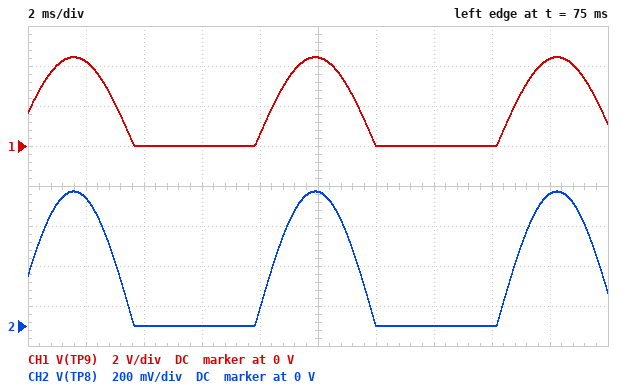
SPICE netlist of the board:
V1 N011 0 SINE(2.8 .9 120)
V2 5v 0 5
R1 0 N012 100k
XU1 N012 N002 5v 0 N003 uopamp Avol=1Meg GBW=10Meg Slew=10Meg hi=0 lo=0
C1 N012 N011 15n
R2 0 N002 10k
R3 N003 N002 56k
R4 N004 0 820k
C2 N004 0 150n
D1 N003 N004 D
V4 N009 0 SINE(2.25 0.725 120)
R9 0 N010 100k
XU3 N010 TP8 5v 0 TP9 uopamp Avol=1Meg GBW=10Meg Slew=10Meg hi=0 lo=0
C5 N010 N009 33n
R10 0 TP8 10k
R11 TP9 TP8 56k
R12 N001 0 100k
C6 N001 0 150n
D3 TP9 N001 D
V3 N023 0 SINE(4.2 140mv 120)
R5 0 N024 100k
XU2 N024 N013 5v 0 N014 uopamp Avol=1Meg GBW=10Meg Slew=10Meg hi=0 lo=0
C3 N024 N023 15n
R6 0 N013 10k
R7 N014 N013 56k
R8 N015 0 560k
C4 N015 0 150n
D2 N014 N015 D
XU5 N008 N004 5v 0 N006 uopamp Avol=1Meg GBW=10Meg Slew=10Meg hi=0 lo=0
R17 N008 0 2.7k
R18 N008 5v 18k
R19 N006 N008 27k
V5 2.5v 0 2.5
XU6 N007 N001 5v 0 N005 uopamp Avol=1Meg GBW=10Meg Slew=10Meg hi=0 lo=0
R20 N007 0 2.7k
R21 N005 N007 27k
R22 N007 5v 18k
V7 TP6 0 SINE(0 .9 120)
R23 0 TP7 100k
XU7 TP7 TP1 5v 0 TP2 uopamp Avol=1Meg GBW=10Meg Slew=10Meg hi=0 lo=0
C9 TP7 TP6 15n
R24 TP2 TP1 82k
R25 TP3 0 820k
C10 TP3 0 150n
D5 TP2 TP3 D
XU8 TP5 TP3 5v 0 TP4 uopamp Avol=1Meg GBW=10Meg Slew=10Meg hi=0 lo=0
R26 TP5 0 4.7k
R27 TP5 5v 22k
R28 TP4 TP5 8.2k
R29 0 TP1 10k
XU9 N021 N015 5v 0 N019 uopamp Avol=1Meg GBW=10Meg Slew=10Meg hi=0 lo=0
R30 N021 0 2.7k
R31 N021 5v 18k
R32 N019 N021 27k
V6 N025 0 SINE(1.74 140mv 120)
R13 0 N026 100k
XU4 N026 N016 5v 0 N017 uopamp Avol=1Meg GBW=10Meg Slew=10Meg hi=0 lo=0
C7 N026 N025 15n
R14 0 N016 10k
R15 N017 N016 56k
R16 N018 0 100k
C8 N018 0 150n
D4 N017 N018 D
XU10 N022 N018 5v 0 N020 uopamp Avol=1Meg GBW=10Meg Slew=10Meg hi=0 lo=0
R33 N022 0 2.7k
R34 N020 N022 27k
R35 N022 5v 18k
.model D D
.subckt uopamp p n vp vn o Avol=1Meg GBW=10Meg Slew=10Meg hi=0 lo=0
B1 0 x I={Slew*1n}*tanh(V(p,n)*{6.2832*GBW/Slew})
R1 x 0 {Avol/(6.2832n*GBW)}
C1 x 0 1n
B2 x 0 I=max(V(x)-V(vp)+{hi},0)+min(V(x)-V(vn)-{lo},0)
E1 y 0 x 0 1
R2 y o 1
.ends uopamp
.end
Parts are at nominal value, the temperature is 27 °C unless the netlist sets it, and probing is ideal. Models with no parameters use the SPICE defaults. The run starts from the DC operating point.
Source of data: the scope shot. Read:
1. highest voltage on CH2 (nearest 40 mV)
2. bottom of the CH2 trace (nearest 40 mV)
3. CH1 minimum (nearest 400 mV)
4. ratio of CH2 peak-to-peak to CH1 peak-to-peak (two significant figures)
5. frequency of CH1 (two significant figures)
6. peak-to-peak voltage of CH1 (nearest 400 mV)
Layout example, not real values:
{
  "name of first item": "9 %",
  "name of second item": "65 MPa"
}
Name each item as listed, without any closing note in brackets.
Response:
{
  "highest voltage on CH2": "680 mV",
  "bottom of the CH2 trace": "0 V",
  "CH1 minimum": "0 V",
  "ratio of CH2 peak-to-peak to CH1 peak-to-peak": "0.15",
  "frequency of CH1": "120 Hz",
  "peak-to-peak voltage of CH1": "4.4 V"
}
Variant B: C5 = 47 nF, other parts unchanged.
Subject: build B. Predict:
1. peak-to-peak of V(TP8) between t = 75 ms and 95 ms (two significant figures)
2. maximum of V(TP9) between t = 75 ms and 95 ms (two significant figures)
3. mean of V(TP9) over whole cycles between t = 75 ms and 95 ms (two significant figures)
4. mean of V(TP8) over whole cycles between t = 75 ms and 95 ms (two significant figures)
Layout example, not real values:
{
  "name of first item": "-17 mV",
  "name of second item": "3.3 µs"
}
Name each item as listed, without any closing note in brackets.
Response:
{
  "peak-to-peak of V(TP8) between t = 75 ms and 95 ms": "700 mV",
  "maximum of V(TP9) between t = 75 ms and 95 ms": "4.6 V",
  "mean of V(TP9) over whole cycles between t = 75 ms and 95 ms": "1.5 V",
  "mean of V(TP8) over whole cycles between t = 75 ms and 95 ms": "220 mV"
}
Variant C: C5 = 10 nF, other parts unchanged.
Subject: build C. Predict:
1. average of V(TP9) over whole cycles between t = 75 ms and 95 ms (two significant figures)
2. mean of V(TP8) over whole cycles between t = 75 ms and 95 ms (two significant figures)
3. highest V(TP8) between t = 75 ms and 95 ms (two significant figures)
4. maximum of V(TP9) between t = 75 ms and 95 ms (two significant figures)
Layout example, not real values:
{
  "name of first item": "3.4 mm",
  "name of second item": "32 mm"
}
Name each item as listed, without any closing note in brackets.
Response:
{
  "average of V(TP9) over whole cycles between t = 75 ms and 95 ms": "910 mV",
  "mean of V(TP8) over whole cycles between t = 75 ms and 95 ms": "140 mV",
  "highest V(TP8) between t = 75 ms and 95 ms": "440 mV",
  "maximum of V(TP9) between t = 75 ms and 95 ms": "2.9 V"
}
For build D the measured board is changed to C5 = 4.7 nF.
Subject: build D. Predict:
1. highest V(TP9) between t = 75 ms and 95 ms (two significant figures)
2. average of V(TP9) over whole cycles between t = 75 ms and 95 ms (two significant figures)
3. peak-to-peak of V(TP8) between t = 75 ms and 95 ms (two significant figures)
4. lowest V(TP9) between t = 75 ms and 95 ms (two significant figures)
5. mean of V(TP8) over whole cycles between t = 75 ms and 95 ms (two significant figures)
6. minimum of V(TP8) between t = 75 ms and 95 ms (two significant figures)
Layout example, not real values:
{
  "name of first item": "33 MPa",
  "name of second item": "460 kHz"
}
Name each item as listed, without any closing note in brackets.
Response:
{
  "highest V(TP9) between t = 75 ms and 95 ms": "1.6 V",
  "average of V(TP9) over whole cycles between t = 75 ms and 95 ms": "510 mV",
  "peak-to-peak of V(TP8) between t = 75 ms and 95 ms": "240 mV",
  "lowest V(TP9) between t = 75 ms and 95 ms": "-9.1 mV",
  "mean of V(TP8) over whole cycles between t = 75 ms and 95 ms": "77 mV",
  "minimum of V(TP8) between t = 75 ms and 95 ms": "-1.4 mV"
}
